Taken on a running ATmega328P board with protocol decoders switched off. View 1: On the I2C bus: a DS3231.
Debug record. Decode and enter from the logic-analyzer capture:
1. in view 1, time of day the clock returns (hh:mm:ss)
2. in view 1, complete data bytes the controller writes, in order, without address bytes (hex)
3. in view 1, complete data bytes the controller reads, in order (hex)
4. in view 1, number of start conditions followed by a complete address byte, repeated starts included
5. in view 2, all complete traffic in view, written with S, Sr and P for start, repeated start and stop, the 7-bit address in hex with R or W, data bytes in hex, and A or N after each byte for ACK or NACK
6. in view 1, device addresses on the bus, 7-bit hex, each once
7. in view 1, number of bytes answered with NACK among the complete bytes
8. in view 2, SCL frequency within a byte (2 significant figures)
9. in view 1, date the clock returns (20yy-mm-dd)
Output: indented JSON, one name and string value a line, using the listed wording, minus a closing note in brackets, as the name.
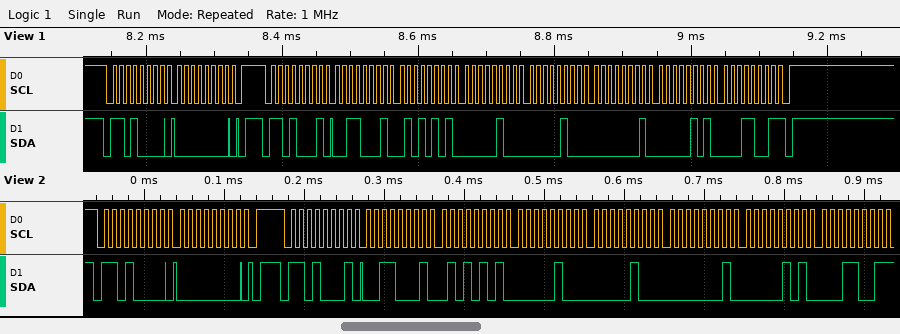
{
  "in view 1, time of day the clock returns": "04:55:31",
  "in view 1, complete data bytes the controller writes, in order, without address bytes": "00",
  "in view 1, complete data bytes the controller reads, in order": "31 55 04 04 01 05 19",
  "in view 1, number of start conditions followed by a complete address byte, repeated starts included": "2",
  "in view 2, all complete traffic in view, written with S, Sr and P for start, repeated start and stop, the 7-bit address in hex with R or W, data bytes in hex, and A or N after each byte for ACK or NACK": "S 68W A 00 A P S 68R A 31 A 55 A 04 A 04 A 01 A 05 A 19 N",
  "in view 1, device addresses on the bus, 7-bit hex, each once": "0x68",
  "in view 1, number of bytes answered with NACK among the complete bytes": "1",
  "in view 2, SCL frequency within a byte": "100 kHz",
  "in view 1, date the clock returns": "2019-05-01"
}
